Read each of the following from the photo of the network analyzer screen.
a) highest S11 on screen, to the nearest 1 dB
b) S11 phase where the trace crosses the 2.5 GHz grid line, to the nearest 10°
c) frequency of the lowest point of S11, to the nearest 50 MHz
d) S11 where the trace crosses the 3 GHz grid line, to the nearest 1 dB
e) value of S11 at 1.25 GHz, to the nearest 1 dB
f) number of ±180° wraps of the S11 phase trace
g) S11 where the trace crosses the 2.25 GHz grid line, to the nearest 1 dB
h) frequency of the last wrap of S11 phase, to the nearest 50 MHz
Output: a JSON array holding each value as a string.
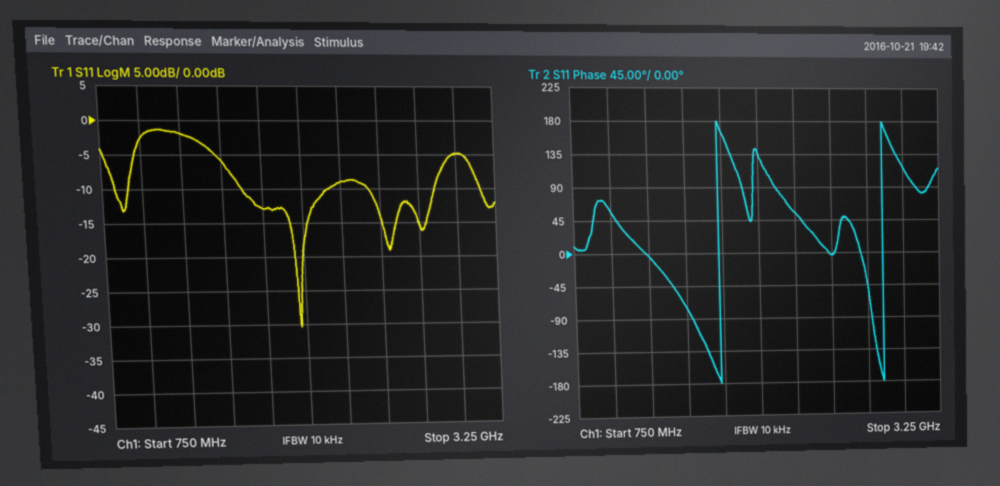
["-1 dB", "0°", "1.95 GHz", "-5 dB", "-2 dB", "2", "-9 dB", "2.85 GHz"]
